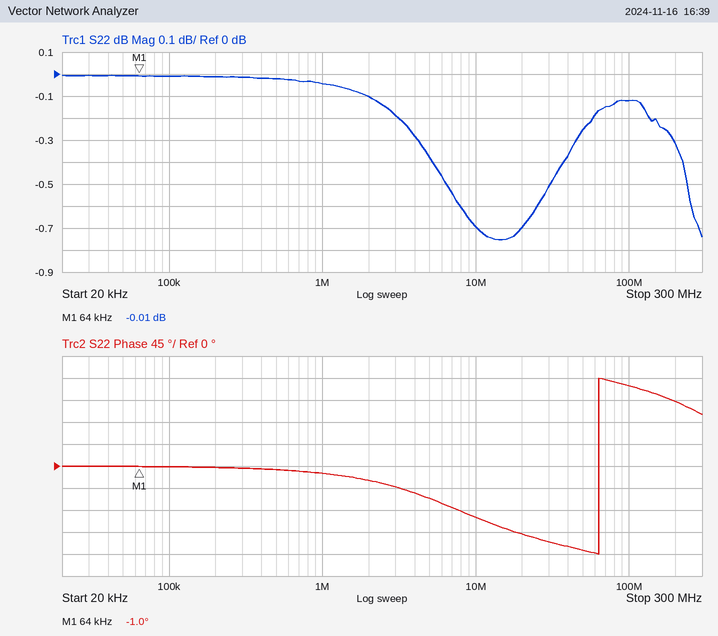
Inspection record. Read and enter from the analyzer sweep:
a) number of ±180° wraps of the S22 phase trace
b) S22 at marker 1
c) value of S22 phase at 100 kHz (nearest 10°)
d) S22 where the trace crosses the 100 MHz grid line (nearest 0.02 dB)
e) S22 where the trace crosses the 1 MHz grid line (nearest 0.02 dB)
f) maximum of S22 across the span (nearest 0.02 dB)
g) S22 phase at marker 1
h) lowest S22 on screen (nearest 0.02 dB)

1
-0.01 dB
0°
-0.12 dB
-0.04 dB
0.00 dB
-1.0°
-0.76 dB
